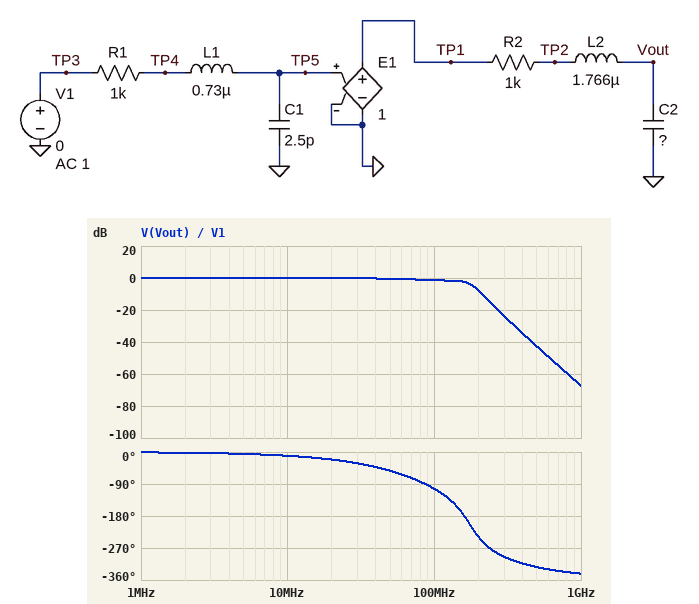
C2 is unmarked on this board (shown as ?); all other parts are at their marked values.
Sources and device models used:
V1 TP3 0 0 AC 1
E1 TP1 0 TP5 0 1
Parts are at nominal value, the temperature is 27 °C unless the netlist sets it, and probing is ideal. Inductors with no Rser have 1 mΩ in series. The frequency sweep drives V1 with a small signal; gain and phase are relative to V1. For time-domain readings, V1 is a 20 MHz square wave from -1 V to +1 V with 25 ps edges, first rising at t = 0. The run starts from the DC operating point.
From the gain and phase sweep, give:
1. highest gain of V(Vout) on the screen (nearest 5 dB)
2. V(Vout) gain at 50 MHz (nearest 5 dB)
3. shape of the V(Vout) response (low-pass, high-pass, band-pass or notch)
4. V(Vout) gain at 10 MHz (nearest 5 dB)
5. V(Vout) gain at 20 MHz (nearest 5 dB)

0 dB
0 dB
low-pass
0 dB
0 dB
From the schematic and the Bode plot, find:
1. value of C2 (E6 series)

470 fF
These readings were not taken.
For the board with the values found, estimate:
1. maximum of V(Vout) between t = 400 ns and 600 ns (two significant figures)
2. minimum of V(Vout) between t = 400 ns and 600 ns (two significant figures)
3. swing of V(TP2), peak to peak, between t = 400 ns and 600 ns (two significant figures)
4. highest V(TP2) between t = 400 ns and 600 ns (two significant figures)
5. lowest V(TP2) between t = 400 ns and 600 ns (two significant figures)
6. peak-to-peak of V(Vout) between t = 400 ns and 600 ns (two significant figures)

1.1 V
-1.1 V
2.0 V
1.0 V
-1.0 V
2.2 V
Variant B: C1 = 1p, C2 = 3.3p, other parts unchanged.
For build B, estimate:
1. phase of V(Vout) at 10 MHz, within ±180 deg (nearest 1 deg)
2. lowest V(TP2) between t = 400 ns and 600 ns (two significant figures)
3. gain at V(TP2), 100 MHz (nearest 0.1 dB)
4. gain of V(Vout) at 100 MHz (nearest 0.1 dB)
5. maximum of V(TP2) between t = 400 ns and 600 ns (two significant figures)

-16 deg
-1.1 V
-5.0 dB
-7.3 dB
1.1 V
